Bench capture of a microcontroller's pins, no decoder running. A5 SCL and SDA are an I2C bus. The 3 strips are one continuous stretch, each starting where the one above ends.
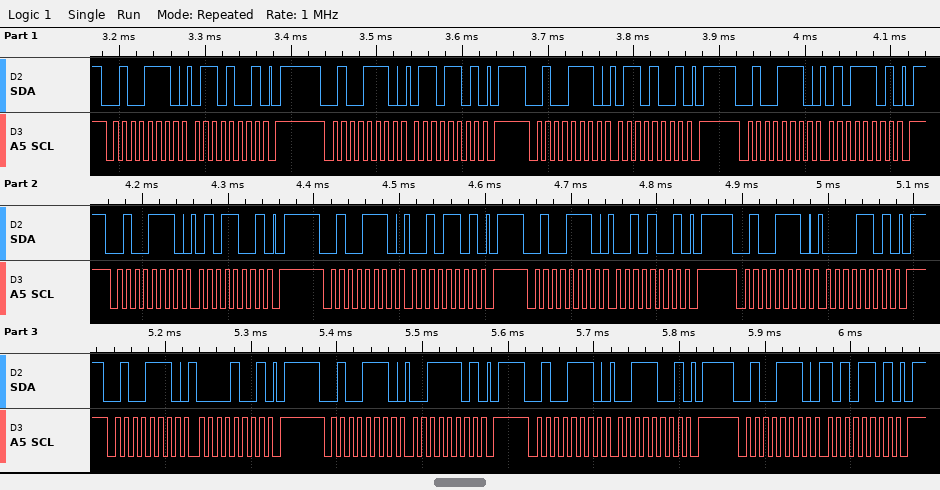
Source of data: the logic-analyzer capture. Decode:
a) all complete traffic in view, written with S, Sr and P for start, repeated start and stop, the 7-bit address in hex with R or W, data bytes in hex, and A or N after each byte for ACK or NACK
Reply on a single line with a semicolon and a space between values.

S 27W A 69 A P S 27W A 6D A P S 27W A 69 A P S 27W A 5D A P S 27W A 59 A P S 27W A 2D A P S 27W A 29 A P S 27W A 0D A P S 27W A 09 A P S 27W A 3D A P S 27W A 39 A P S 27W A AD A P
